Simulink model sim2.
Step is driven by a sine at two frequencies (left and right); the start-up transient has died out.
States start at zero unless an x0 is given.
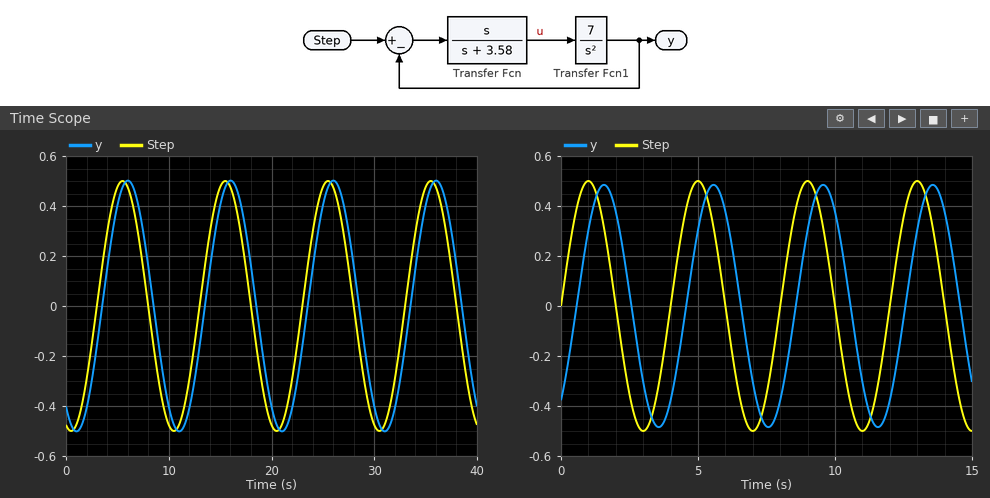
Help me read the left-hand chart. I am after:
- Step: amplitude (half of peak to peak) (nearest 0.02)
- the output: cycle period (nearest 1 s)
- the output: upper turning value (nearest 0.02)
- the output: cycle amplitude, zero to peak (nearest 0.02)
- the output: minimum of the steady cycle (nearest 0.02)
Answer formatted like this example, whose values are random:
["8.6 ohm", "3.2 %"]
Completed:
["0.50", "10 s", "0.50", "0.50", "-0.50"]
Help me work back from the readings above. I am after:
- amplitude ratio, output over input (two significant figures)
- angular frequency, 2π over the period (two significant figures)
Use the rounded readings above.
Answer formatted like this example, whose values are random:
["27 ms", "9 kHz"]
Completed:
["1.0", "0.63 rad/s"]
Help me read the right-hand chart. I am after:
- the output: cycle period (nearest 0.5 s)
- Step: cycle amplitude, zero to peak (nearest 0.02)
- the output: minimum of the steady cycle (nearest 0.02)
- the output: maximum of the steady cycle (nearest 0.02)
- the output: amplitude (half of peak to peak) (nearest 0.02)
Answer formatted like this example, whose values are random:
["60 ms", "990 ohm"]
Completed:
["4.0 s", "0.50", "-0.48", "0.48", "0.48"]
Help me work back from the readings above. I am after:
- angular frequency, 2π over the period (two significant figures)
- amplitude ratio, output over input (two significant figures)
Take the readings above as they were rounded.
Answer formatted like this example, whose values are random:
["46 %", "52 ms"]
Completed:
["1.6 rad/s", "0.96"]
